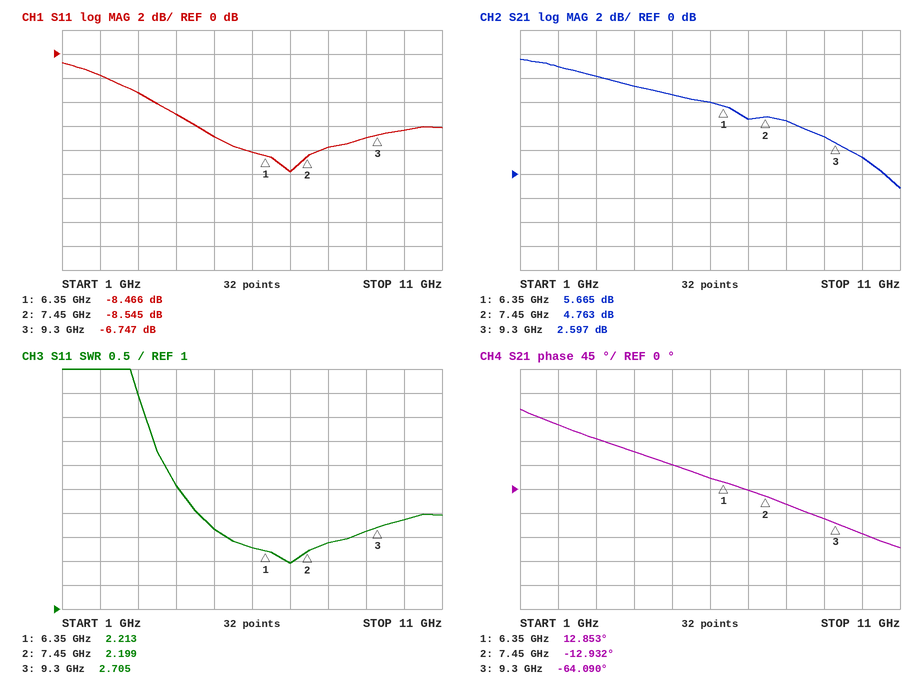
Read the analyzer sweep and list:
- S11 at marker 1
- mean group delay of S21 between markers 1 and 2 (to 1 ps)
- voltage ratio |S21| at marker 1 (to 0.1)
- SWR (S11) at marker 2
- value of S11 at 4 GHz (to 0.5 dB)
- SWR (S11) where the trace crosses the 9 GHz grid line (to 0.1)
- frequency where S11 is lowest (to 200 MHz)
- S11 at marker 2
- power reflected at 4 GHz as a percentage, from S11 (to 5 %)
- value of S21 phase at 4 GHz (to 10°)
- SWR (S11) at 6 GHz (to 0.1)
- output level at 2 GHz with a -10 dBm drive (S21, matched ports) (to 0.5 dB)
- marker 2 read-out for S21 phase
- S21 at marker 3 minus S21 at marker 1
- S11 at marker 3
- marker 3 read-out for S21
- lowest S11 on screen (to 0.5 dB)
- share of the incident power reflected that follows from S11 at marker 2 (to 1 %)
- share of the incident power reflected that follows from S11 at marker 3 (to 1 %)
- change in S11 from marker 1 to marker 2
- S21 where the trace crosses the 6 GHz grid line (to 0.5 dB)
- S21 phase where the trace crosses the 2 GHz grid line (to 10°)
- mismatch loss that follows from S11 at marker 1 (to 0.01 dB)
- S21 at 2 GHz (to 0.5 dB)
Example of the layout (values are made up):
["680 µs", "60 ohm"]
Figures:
["-8.466 dB", "65 ps", "1.9", "2.199", "-5.0 dB", "2.6", "7.0 GHz", "-8.545 dB", "30 %", "70°", "2.3", "-1.0 dBm", "-12.932°", "-3.068 dB", "-6.747 dB", "2.597 dB", "-10.0 dB", "14 %", "21 %", "-0.079 dB", "6.0 dB", "120°", "0.67 dB", "9.0 dB"]
